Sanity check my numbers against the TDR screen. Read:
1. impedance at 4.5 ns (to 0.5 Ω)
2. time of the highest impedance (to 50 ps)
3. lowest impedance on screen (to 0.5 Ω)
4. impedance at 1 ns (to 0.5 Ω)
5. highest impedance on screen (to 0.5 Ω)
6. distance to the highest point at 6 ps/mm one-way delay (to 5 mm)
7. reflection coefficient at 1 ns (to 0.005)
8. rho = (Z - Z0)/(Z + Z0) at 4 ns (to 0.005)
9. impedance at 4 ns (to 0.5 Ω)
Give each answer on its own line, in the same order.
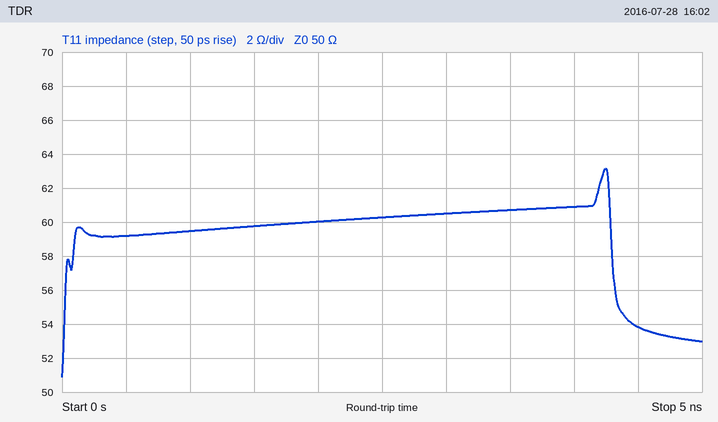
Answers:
54.0 Ω
4.25 ns
51.0 Ω
59.5 Ω
63.0 Ω
355 mm
+0.085
+0.100
61.0 Ω
